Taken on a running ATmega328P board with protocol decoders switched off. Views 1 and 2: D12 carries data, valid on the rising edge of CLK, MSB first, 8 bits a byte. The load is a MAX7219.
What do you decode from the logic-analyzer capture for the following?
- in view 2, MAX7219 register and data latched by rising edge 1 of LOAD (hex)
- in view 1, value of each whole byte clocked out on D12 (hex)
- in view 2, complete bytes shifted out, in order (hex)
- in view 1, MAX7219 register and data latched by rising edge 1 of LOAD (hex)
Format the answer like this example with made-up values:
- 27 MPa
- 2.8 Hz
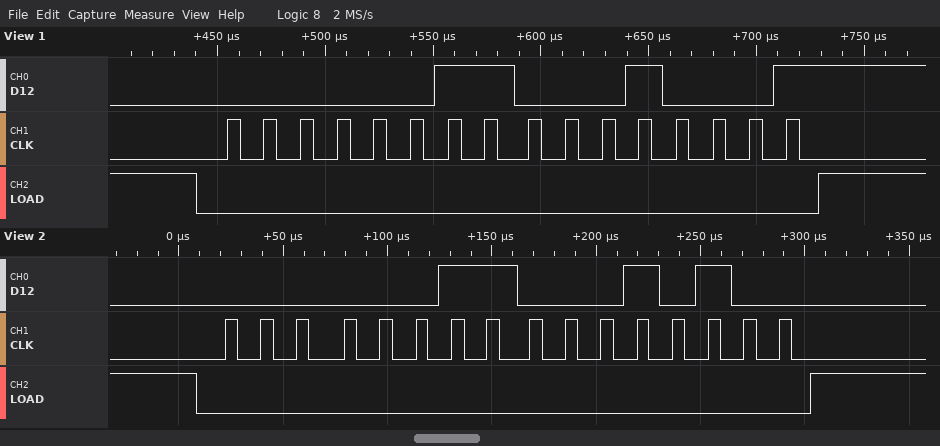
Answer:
- register 0x3, data 0x14
- 0x03 0x11
- 03 14
- register 0x3, data 0x11
